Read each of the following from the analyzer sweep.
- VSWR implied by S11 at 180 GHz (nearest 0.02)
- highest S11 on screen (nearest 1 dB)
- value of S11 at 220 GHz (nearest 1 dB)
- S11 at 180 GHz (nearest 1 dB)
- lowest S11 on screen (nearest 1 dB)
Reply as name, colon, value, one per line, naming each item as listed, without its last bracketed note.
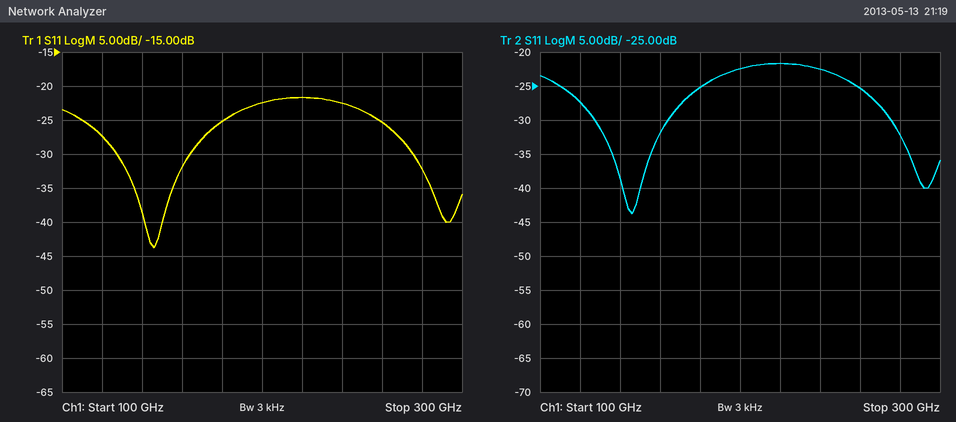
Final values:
VSWR implied by S11 at 180 GHz: 1.12
highest S11 on screen: -22 dB
value of S11 at 220 GHz: -22 dB
S11 at 180 GHz: -25 dB
lowest S11 on screen: -44 dB
